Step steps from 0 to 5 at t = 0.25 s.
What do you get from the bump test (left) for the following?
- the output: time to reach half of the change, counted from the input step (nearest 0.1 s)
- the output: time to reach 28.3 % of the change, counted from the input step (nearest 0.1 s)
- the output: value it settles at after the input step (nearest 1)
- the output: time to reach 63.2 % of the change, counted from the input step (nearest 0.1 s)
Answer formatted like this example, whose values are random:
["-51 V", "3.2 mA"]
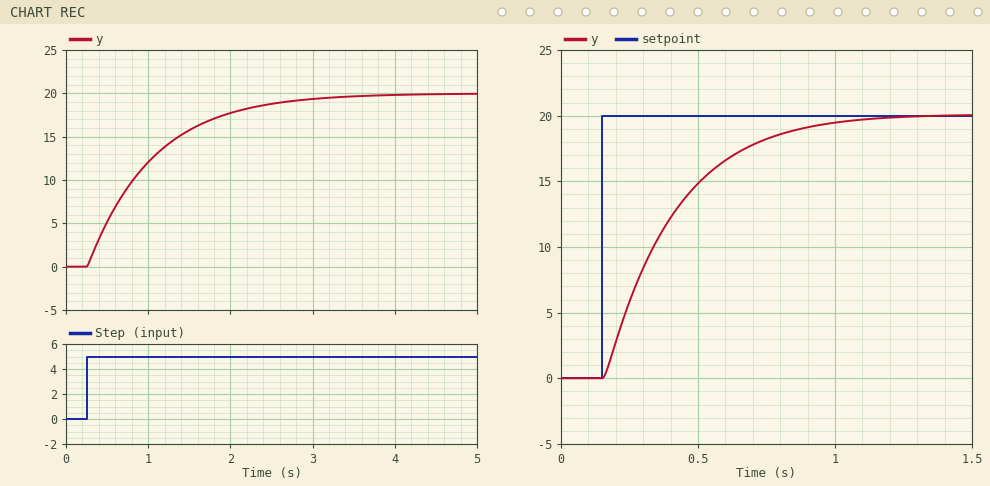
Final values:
["0.6 s", "0.3 s", "20", "0.8 s"]
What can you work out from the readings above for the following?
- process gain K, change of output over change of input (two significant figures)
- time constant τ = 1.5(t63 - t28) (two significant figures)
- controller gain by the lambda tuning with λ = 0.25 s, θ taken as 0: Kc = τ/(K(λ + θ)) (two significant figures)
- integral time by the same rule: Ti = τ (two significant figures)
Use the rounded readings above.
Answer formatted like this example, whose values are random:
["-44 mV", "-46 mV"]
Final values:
["4.0", "0.75 s", "0.75", "0.75 s"]
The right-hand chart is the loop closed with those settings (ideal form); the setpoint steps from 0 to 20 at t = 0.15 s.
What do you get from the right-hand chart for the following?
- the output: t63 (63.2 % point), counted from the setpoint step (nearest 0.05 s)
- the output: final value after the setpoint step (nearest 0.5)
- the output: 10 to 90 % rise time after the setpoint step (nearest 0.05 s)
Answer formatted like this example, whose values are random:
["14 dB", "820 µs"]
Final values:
["0.25 s", "20.0", "0.55 s"]
